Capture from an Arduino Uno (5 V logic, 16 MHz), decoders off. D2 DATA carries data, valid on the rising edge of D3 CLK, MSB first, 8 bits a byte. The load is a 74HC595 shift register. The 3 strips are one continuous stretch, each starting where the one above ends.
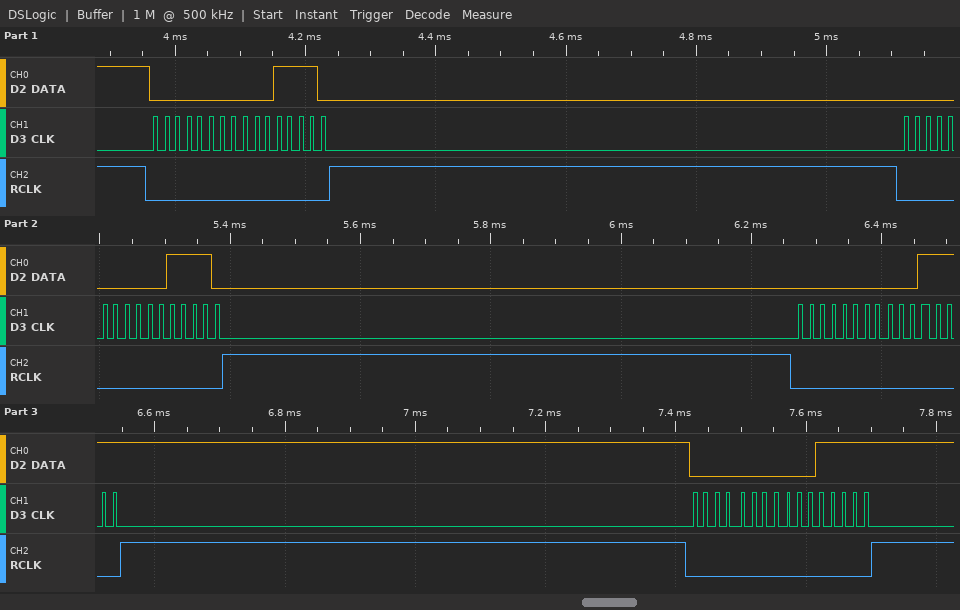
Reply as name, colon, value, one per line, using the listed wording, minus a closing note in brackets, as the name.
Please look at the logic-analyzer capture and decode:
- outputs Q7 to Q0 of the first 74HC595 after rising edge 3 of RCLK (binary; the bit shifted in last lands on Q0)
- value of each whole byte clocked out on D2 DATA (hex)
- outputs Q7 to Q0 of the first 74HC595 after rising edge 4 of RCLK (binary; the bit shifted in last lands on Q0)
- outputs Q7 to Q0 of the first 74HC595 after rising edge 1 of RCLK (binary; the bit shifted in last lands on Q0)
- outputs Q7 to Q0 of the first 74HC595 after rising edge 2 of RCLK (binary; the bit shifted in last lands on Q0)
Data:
outputs Q7 to Q0 of the first 74HC595 after rising edge 3 of RCLK: 00011111
value of each whole byte clocked out on D2 DATA: 00 1E 00 1E 00 1F 00 1F
outputs Q7 to Q0 of the first 74HC595 after rising edge 4 of RCLK: 00011111
outputs Q7 to Q0 of the first 74HC595 after rising edge 1 of RCLK: 00011110
outputs Q7 to Q0 of the first 74HC595 after rising edge 2 of RCLK: 00011110
